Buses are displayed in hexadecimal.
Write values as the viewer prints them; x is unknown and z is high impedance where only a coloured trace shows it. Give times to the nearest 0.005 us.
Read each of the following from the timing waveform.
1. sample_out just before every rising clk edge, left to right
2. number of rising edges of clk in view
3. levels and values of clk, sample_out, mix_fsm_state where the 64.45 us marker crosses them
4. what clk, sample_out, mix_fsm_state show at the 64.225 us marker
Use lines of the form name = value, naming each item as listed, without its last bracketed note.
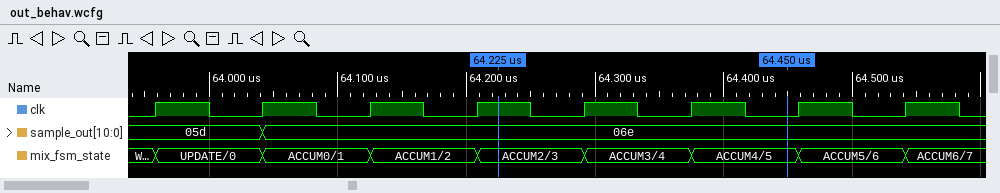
sample_out just before every rising clk edge, left to right = 05d, 05d, 06e, 06e, 06e, 06e, 06e, 06e
number of rising edges of clk in view = 8
levels and values of clk, sample_out, mix_fsm_state where the 64.45 us marker crosses them = clk=0, sample_out=06e, mix_fsm_state=ACCUM4/5
what clk, sample_out, mix_fsm_state show at the 64.225 us marker = clk=1, sample_out=06e, mix_fsm_state=ACCUM2/3
